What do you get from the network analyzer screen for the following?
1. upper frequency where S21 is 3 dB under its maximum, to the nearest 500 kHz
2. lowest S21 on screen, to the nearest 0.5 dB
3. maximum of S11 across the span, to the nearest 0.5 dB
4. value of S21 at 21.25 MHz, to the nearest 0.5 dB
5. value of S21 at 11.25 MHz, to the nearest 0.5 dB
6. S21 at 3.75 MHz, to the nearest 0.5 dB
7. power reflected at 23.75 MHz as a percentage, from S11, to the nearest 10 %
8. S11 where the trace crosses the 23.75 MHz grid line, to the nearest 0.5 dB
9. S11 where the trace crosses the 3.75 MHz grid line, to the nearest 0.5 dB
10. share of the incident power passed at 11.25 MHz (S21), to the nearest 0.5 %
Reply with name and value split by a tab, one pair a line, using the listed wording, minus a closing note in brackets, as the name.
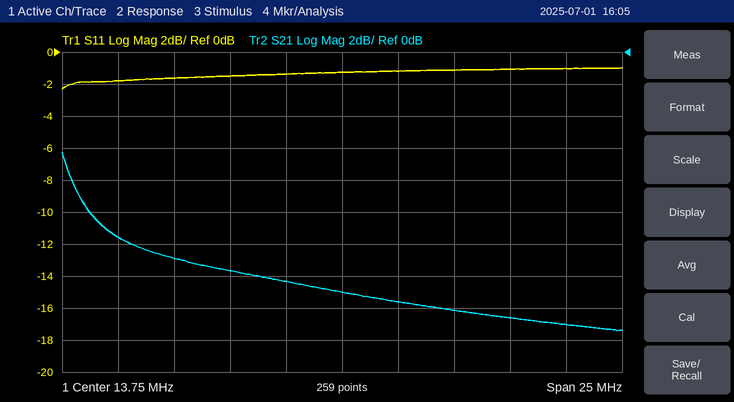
upper frequency where S21 is 3 dB under its maximum, to the nearest 500 kHz	2.0 MHz
lowest S21 on screen, to the nearest 0.5 dB	-17.5 dB
maximum of S11 across the span, to the nearest 0.5 dB	-1.0 dB
value of S21 at 21.25 MHz, to the nearest 0.5 dB	-16.5 dB
value of S21 at 11.25 MHz, to the nearest 0.5 dB	-14.5 dB
S21 at 3.75 MHz, to the nearest 0.5 dB	-11.5 dB
power reflected at 23.75 MHz as a percentage, from S11, to the nearest 10 %	80 %
S11 where the trace crosses the 23.75 MHz grid line, to the nearest 0.5 dB	-1.0 dB
S11 where the trace crosses the 3.75 MHz grid line, to the nearest 0.5 dB	-2.0 dB
share of the incident power passed at 11.25 MHz (S21), to the nearest 0.5 %	3.5 %
